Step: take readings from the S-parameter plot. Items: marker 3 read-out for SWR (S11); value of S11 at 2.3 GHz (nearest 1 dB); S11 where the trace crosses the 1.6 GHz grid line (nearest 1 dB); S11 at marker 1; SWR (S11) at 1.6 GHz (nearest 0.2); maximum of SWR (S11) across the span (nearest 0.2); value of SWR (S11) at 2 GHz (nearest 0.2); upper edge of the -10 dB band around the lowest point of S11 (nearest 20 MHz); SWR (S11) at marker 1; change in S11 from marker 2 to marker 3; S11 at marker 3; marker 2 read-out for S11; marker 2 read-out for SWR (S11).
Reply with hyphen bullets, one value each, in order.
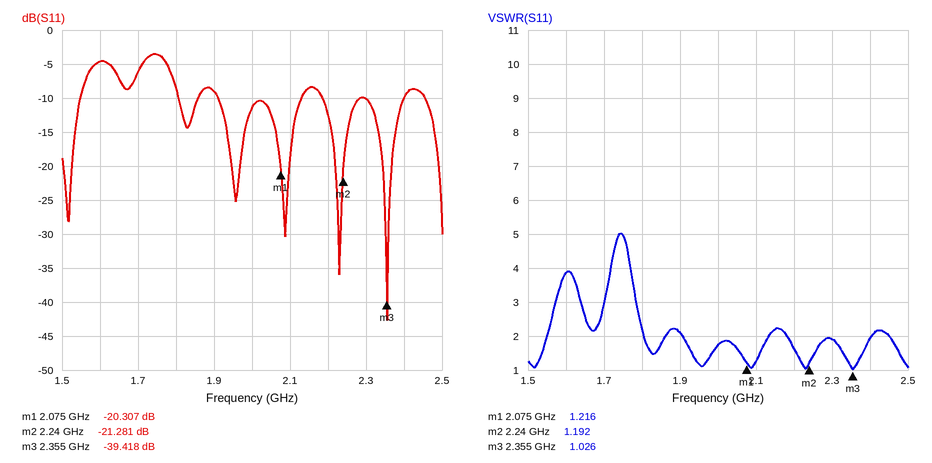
- 1.026
- -10 dB
- -5 dB
- -20.307 dB
- 3.8
- 5.0
- 1.8
- 2.40 GHz
- 1.216
- -18.137 dB
- -39.418 dB
- -21.281 dB
- 1.192
